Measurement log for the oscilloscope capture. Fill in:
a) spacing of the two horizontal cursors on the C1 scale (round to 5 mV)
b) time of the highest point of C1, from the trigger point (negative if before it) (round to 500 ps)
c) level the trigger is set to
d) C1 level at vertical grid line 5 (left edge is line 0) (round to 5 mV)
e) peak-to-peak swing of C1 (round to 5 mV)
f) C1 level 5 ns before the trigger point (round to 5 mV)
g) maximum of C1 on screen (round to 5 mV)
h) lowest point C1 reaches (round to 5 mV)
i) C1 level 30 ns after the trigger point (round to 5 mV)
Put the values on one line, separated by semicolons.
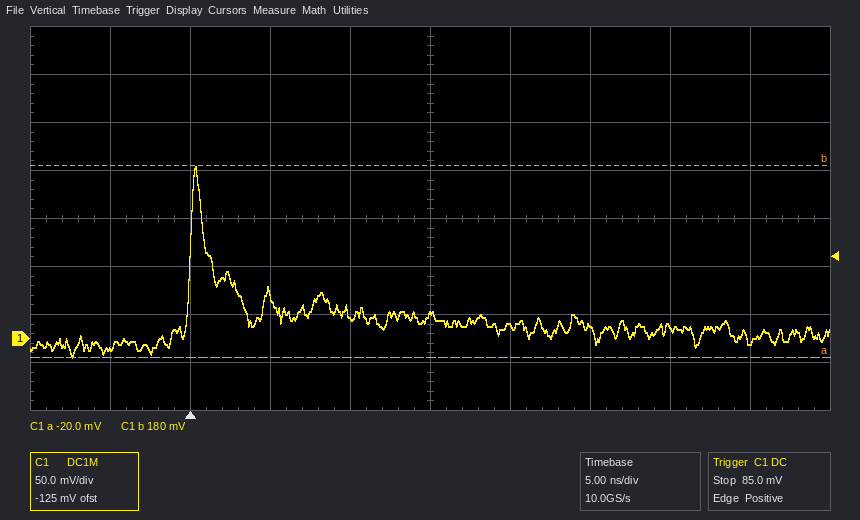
200 mV; +500 ps; 85.0 mV; 25 mV; 200 mV; -10 mV; 180 mV; -20 mV; 10 mV
